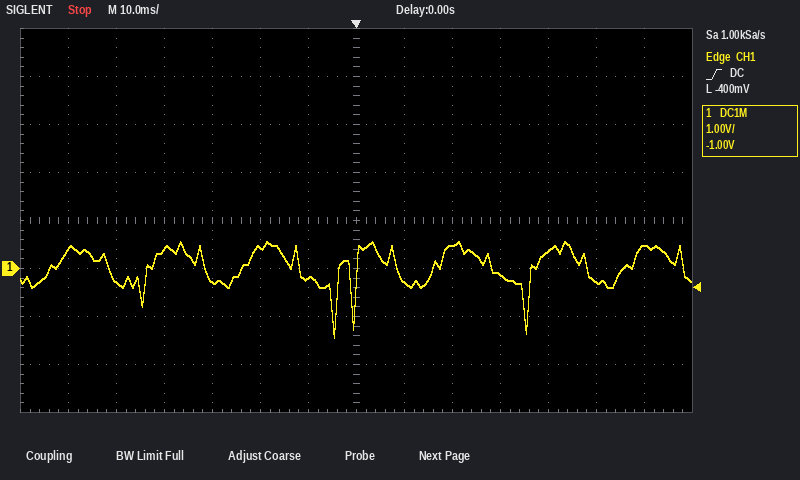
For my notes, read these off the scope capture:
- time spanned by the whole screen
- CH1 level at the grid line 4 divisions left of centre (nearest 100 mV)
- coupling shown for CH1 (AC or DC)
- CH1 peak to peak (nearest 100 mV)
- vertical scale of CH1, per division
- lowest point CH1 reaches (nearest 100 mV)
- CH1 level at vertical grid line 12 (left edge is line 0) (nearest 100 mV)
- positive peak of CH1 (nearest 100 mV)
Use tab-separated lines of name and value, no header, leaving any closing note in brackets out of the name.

time spanned by the whole screen	140 ms
CH1 level at the grid line 4 divisions left of centre	400 mV
coupling shown for CH1	DC
CH1 peak to peak	2.0 V
vertical scale of CH1, per division	1 V
lowest point CH1 reaches	-1.4 V
CH1 level at vertical grid line 12 (left edge is line 0)	-300 mV
positive peak of CH1	600 mV
